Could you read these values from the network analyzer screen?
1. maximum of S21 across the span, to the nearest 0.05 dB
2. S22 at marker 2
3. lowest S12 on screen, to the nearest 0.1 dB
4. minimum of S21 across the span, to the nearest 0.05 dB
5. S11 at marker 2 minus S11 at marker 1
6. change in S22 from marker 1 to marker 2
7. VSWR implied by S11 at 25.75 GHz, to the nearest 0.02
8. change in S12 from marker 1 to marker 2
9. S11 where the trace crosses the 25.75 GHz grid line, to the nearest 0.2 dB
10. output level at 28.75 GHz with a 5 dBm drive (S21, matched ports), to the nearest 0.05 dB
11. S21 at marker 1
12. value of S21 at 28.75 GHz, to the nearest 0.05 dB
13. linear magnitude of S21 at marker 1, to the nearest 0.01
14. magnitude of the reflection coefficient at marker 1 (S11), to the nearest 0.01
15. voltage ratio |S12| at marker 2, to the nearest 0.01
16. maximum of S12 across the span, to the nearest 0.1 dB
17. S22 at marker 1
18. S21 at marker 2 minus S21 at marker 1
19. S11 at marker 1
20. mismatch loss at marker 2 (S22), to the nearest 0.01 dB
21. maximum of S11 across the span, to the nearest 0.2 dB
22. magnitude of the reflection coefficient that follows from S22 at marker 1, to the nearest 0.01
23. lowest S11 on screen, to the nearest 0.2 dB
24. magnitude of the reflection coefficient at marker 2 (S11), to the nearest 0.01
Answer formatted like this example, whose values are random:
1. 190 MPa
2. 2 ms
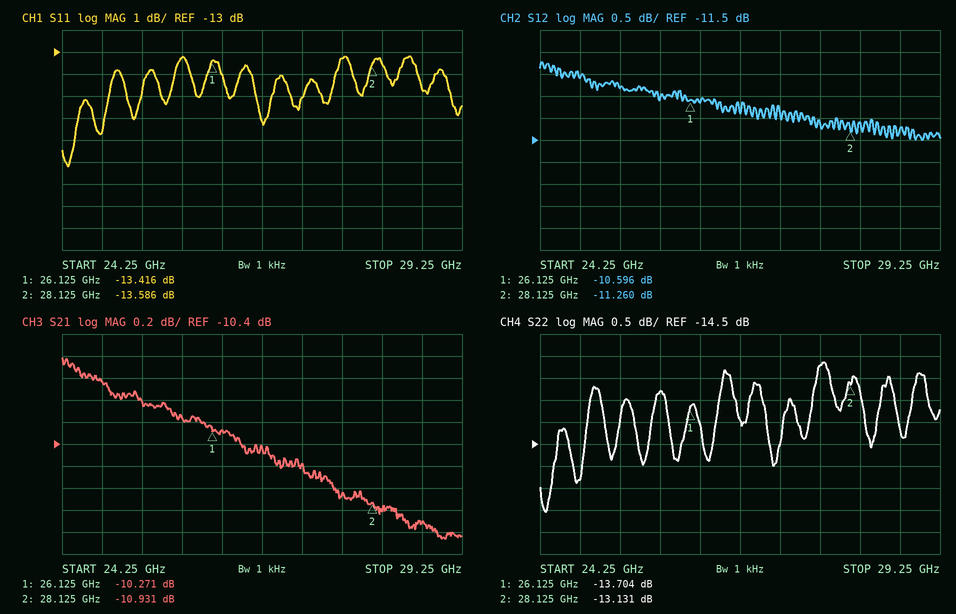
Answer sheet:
1. -9.60 dB
2. -13.131 dB
3. -11.5 dB
4. -11.25 dB
5. -0.170 dB
6. 0.573 dB
7. 1.56
8. -0.664 dB
9. -13.2 dB
10. -6.10 dBm
11. -10.271 dB
12. -11.10 dB
13. 0.31
14. 0.21
15. 0.27
16. -9.7 dB
17. -13.704 dB
18. -0.660 dB
19. -13.416 dB
20. 0.22 dB
21. -13.2 dB
22. 0.21
23. -18.2 dB
24. 0.21
